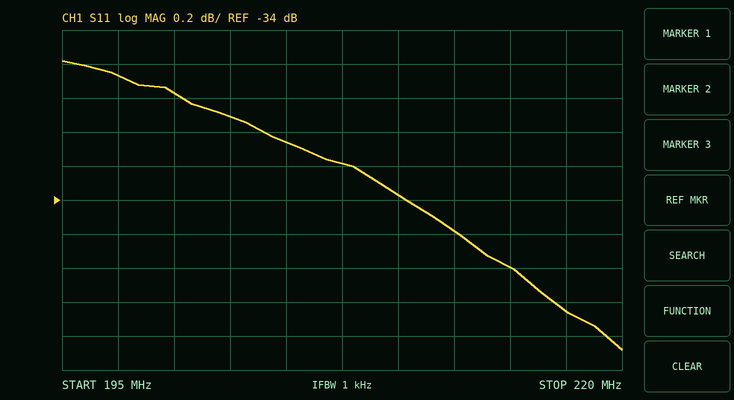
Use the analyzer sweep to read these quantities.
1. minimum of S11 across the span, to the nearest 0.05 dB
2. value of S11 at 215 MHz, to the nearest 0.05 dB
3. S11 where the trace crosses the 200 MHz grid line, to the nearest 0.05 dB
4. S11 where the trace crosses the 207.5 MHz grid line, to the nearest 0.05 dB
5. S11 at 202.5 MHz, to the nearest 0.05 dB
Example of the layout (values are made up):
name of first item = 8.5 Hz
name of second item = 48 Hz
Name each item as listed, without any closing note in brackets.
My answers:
minimum of S11 across the span, to the nearest 0.05 dB = -34.90 dB
value of S11 at 215 MHz, to the nearest 0.05 dB = -34.40 dB
S11 where the trace crosses the 200 MHz grid line, to the nearest 0.05 dB = -33.35 dB
S11 where the trace crosses the 207.5 MHz grid line, to the nearest 0.05 dB = -33.80 dB
S11 at 202.5 MHz, to the nearest 0.05 dB = -33.50 dB
